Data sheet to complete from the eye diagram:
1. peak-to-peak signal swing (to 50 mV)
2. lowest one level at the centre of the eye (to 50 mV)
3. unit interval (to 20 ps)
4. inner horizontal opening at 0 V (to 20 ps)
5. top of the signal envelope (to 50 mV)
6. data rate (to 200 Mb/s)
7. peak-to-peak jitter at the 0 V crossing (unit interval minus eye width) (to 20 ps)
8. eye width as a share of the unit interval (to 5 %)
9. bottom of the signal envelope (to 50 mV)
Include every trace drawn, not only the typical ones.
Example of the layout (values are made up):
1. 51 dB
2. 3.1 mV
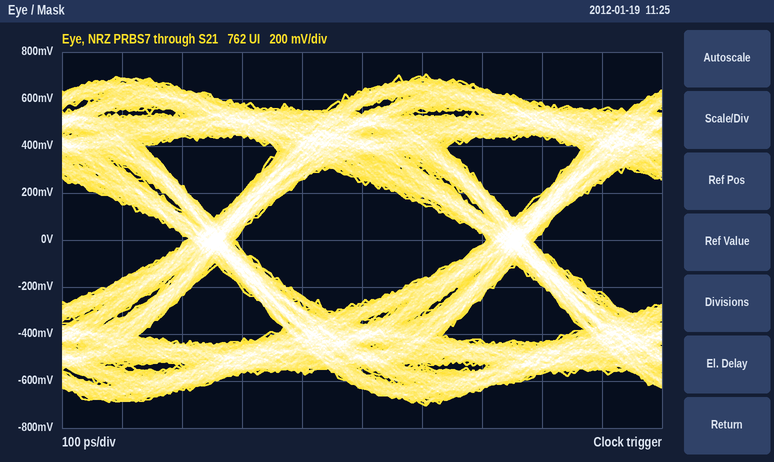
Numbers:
1. 1.40 V
2. 250 mV
3. 500 ps
4. 420 ps
5. 700 mV
6. 2.0 Gb/s
7. 80 ps
8. 85 %
9. -700 mV
